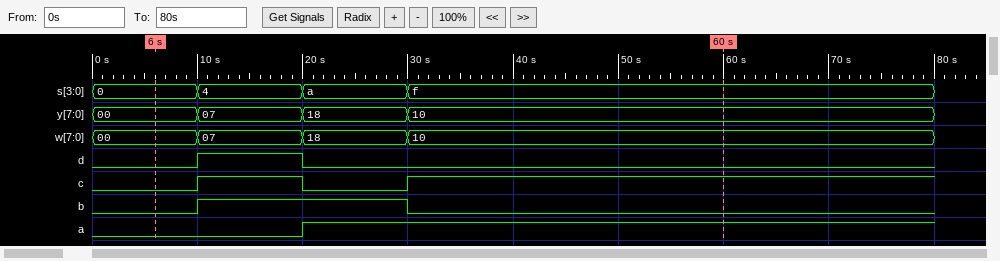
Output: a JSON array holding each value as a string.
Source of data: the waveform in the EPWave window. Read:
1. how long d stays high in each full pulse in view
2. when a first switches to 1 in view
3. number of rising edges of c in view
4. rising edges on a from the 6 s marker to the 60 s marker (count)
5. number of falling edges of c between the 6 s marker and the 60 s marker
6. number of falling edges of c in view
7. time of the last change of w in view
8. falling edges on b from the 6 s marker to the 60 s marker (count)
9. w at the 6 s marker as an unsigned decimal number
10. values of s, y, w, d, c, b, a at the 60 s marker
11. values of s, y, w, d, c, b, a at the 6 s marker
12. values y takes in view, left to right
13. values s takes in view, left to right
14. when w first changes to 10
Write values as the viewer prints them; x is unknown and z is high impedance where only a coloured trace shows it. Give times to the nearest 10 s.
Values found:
["10 s", "20 s", "2", "1", "1", "1", "30 s", "1", "0", "s=f, y=10, w=10, d=0, c=1, b=0, a=1", "s=0, y=00, w=00, d=0, c=0, b=0, a=0", "00, 07, 18, 10", "0, 4, a, f", "30 s"]
